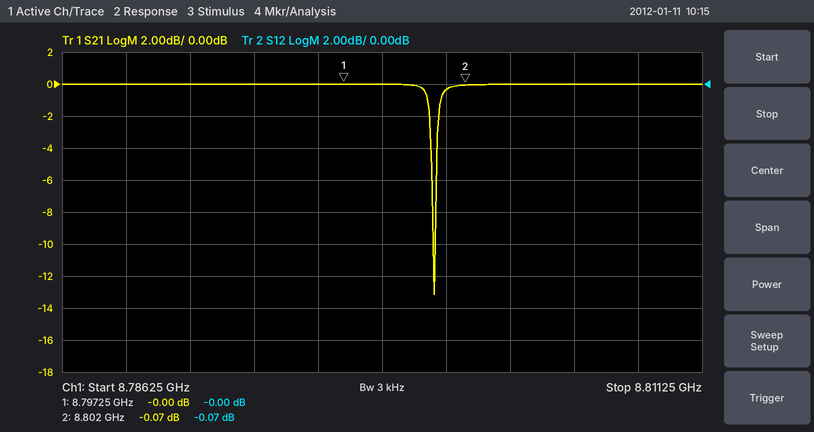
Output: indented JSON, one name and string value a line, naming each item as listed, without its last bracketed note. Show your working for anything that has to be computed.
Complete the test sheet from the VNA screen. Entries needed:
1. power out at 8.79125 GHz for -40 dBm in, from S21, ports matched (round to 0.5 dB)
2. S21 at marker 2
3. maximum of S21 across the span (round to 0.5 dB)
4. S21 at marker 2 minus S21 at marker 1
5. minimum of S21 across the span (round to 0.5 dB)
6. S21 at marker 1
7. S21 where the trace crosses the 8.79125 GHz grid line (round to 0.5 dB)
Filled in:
{
  "power out at 8.79125 GHz for -40 dBm in, from S21, ports matched": "-40 dBm + (0.0 dB) = -40.0 dBm",
  "S21 at marker 2": "-0.07 dB",
  "maximum of S21 across the span": "0.0 dB",
  "S21 at marker 2 minus S21 at marker 1": "-0.07 − (-0) = -0.07 dB",
  "minimum of S21 across the span": "-13.0 dB",
  "S21 at marker 1": "-0.00 dB",
  "S21 where the trace crosses the 8.79125 GHz grid line": "0.0 dB"
}
